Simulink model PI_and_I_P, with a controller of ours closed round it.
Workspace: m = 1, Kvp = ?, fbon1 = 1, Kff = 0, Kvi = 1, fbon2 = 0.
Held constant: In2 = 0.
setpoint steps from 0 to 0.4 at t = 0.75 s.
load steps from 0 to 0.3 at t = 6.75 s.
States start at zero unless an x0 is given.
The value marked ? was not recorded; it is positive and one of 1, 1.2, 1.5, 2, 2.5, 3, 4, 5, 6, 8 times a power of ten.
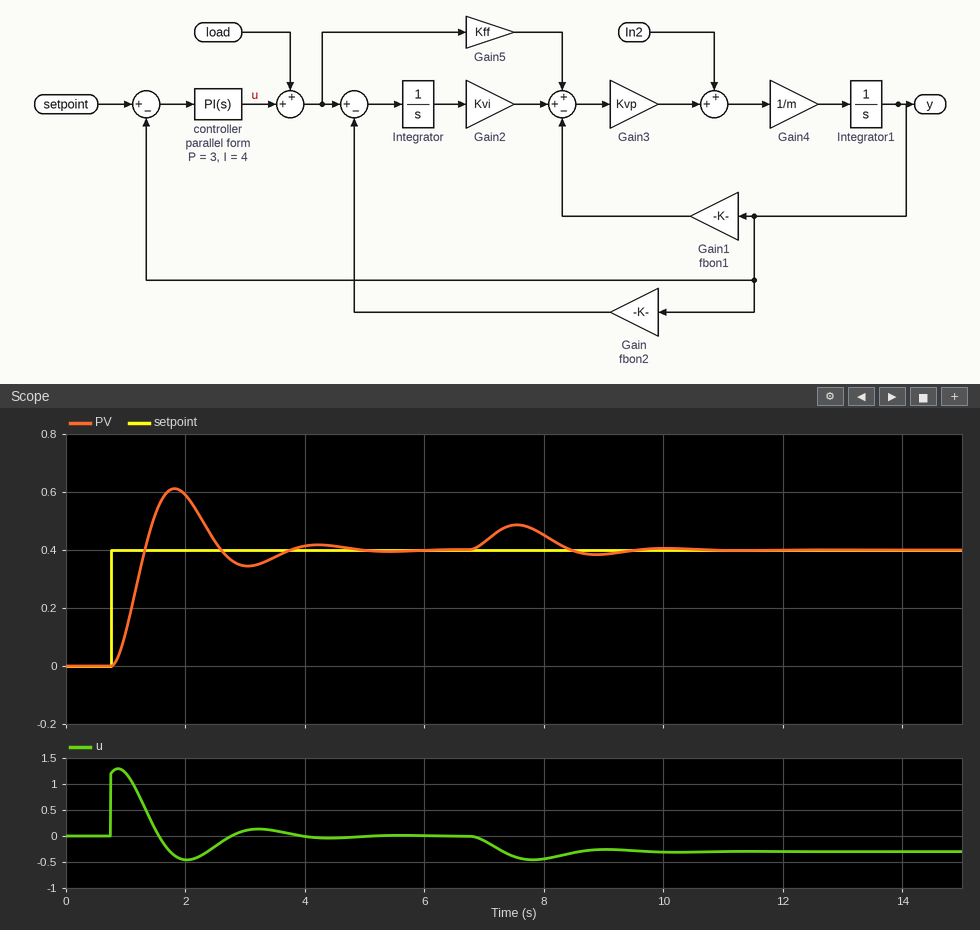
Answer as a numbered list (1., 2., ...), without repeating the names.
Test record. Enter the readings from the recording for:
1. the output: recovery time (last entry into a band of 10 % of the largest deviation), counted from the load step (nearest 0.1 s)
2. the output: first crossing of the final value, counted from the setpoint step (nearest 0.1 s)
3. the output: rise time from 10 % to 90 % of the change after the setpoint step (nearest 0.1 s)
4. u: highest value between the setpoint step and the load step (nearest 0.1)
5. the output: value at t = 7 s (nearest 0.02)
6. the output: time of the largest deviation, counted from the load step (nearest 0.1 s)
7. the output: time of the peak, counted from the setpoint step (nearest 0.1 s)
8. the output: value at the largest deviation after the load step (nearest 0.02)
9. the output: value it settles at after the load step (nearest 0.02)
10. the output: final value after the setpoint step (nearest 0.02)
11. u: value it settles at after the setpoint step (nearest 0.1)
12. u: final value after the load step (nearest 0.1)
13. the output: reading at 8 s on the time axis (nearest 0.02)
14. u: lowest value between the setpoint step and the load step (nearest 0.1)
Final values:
1. 2.5 s
2. 0.6 s
3. 0.4 s
4. 1.3
5. 0.42
6. 0.8 s
7. 1.1 s
8. 0.48
9. 0.40
10. 0.40
11. 0.0
12. -0.3
13. 0.46
14. -0.5
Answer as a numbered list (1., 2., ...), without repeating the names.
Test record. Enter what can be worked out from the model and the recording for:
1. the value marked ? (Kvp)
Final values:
1. 4
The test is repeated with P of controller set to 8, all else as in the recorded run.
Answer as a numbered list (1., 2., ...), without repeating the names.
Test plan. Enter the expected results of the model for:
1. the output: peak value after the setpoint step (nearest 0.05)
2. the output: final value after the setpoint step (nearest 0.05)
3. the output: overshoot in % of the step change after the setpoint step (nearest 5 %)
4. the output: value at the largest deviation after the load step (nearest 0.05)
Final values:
1. 0.55
2. 0.40
3. 40 %
4. 0.45
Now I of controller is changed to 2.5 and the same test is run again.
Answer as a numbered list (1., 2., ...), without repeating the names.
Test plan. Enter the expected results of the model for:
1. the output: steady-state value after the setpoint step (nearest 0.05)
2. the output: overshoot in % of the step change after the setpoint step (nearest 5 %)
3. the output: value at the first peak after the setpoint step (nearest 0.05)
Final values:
1. 0.40
2. 40 %
3. 0.55
